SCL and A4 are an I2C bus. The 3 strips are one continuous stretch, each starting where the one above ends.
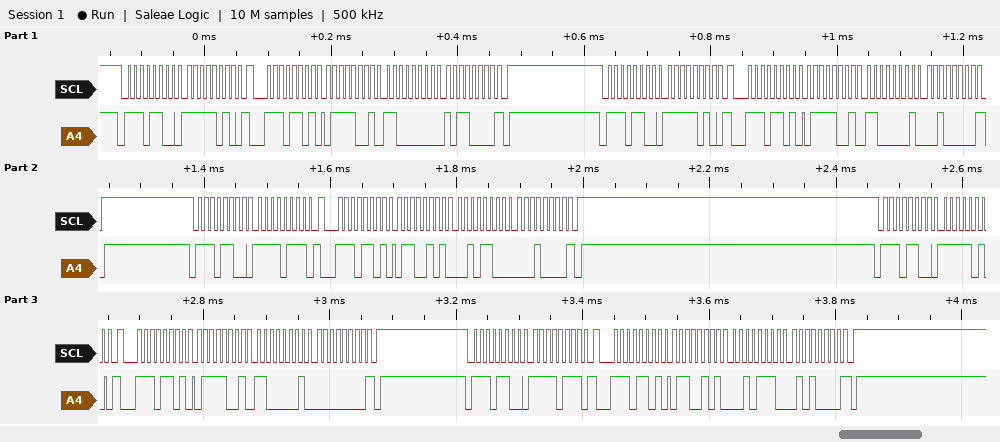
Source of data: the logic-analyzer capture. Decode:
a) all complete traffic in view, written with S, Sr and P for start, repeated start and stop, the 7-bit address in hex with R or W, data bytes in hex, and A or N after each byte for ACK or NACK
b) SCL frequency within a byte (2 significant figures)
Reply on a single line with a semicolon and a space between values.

S 76W A FA A Sr 76R A 79 A C0 A B0 N P S 76W A FA A Sr 76R A 79 A C1 A 20 N P S 76W A F7 A Sr 76R A 65 A 2C A 10 N P S 76W A FA A Sr 76R A 79 A C1 A 00 N P S 76W A F7 A Sr 76R A 65 A 2E A 50 N P; 100 kHz
